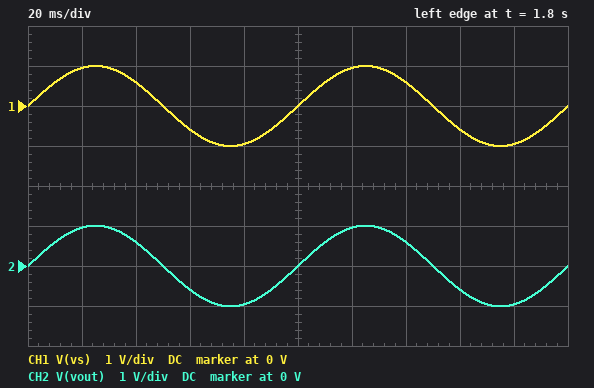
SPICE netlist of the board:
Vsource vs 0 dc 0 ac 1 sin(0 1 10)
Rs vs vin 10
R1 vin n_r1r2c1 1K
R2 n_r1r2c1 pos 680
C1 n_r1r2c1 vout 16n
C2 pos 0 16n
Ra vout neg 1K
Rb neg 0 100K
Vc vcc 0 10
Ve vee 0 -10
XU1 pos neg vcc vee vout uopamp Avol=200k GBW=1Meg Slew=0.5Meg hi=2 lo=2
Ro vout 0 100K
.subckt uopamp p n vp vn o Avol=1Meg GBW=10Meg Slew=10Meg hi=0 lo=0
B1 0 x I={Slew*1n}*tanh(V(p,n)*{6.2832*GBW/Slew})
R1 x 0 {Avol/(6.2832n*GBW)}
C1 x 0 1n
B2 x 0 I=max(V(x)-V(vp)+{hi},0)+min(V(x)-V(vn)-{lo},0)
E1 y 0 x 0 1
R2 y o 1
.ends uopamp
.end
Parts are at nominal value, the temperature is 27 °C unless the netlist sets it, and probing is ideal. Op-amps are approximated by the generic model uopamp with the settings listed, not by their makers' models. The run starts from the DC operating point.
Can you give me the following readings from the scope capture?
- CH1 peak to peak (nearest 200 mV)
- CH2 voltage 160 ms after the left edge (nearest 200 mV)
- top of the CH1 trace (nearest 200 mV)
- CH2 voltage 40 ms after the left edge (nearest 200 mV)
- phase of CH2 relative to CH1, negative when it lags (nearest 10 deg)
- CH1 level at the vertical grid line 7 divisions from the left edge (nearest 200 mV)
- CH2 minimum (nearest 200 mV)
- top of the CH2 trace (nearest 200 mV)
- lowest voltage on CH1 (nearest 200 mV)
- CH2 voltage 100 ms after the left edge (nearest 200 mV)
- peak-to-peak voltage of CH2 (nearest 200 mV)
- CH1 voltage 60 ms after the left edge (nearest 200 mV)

2.0 V
-600 mV
1.0 V
600 mV
0 deg
600 mV
-1.0 V
1.0 V
-1.0 V
0 V
2.0 V
-600 mV
